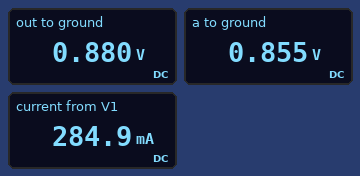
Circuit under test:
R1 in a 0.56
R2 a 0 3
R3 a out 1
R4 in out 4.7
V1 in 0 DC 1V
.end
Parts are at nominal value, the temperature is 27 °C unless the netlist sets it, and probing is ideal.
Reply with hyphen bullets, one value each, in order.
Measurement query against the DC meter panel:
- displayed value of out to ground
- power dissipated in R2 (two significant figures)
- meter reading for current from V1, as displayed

- 0.880 V
- 240 mW
- 284.9 mA
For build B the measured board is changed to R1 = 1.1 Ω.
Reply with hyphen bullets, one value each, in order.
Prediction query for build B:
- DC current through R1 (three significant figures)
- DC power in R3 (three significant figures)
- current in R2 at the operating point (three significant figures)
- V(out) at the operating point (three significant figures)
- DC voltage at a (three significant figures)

- 214 mA
- 1.70 mW
- 255 mA
- 806 mV
- 765 mV
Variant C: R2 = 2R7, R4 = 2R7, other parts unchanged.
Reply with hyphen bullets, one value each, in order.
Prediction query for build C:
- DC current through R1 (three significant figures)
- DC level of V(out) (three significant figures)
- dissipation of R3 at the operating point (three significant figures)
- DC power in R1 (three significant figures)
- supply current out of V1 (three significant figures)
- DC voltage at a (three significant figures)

- 273 mA
- 889 mV
- 1.70 mW
- 41.6 mW
- 314 mA
- 847 mV
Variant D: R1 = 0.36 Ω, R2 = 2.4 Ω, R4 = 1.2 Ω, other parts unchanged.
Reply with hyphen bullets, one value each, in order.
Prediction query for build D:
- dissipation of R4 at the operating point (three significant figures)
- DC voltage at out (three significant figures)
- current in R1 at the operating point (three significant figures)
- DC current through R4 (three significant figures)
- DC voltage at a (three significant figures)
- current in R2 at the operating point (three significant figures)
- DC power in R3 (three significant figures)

- 3.23 mW
- 938 mV
- 317 mA
- 51.9 mA
- 886 mV
- 369 mA
- 2.69 mW
